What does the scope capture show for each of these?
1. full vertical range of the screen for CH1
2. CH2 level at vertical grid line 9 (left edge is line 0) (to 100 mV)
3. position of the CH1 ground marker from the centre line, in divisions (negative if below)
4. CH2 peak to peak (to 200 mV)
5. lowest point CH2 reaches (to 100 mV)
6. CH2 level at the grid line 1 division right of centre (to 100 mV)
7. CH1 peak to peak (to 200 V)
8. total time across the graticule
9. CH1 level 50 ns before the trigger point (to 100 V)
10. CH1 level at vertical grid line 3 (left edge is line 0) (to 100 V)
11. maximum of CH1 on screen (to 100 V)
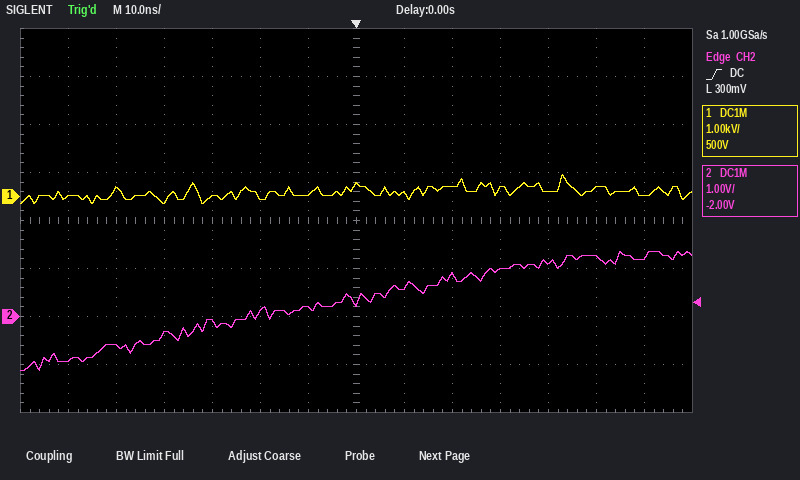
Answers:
8 kV
900 mV
+0.5 div
2.4 V
-1.1 V
600 mV
600 V
140 ns
200 V
-100 V
500 V
